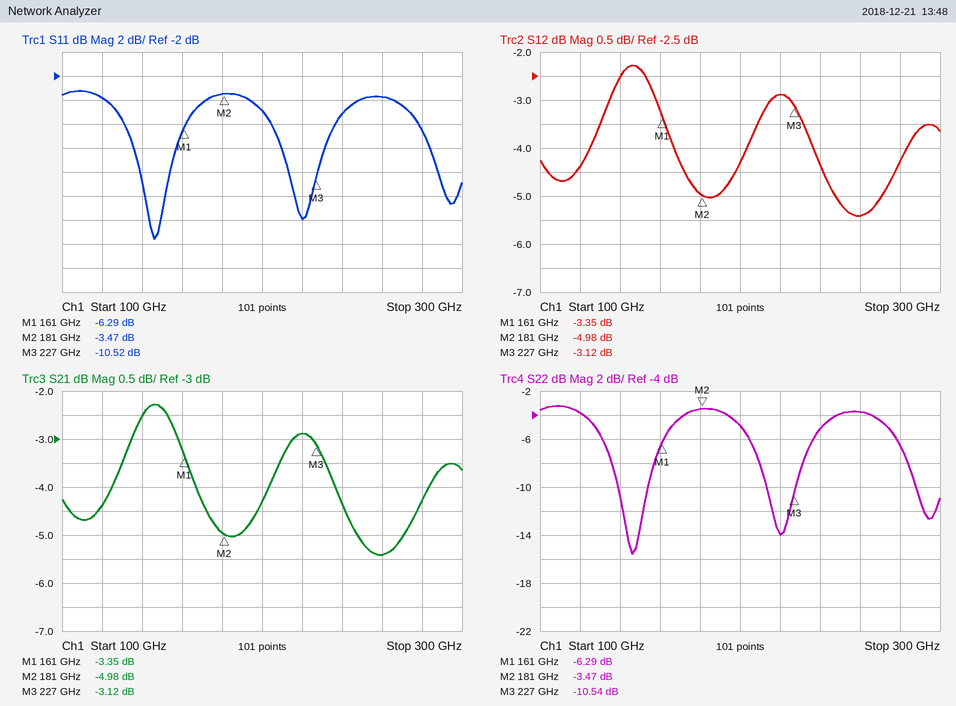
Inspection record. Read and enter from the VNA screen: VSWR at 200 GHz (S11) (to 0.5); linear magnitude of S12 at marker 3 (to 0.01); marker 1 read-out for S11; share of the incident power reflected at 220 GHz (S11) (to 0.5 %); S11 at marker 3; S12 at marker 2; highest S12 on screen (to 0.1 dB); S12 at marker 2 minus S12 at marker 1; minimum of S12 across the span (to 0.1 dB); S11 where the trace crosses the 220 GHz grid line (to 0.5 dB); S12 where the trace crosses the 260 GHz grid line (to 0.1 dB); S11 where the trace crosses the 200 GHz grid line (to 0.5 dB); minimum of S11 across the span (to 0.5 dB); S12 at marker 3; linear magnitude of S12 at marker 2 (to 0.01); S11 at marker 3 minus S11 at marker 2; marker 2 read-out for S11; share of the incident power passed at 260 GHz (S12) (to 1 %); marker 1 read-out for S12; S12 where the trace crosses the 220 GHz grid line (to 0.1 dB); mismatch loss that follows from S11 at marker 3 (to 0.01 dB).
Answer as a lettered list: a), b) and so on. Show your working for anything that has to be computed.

a) |Γ| = 10^(-5/20) = 0.5623; VSWR = (1 + 0.5623)/(1 − 0.5623) ≈ 3.57, so 3.5 to the nearest 0.5
b) 10^(-3.12/20) ≈ 0.70
c) -6.29 dB
d) 10^(-14/10) ≈ 4.0 %
e) -10.52 dB
f) -4.98 dB
g) -2.3 dB
h) -4.98 − (-3.35) = -1.63 dB
i) -5.4 dB
j) -14.0 dB
k) -5.4 dB
l) -5.0 dB
m) -15.5 dB
n) -3.12 dB
o) 10^(-4.98/20) ≈ 0.56
p) -10.52 − (-3.47) = -7.05 dB
q) -3.47 dB
r) 10^(-5.4/10) ≈ 29 %
s) -3.35 dB
t) -2.9 dB
u) −10 log10(1 − 10^(-10.52/10)) ≈ 0.40 dB
